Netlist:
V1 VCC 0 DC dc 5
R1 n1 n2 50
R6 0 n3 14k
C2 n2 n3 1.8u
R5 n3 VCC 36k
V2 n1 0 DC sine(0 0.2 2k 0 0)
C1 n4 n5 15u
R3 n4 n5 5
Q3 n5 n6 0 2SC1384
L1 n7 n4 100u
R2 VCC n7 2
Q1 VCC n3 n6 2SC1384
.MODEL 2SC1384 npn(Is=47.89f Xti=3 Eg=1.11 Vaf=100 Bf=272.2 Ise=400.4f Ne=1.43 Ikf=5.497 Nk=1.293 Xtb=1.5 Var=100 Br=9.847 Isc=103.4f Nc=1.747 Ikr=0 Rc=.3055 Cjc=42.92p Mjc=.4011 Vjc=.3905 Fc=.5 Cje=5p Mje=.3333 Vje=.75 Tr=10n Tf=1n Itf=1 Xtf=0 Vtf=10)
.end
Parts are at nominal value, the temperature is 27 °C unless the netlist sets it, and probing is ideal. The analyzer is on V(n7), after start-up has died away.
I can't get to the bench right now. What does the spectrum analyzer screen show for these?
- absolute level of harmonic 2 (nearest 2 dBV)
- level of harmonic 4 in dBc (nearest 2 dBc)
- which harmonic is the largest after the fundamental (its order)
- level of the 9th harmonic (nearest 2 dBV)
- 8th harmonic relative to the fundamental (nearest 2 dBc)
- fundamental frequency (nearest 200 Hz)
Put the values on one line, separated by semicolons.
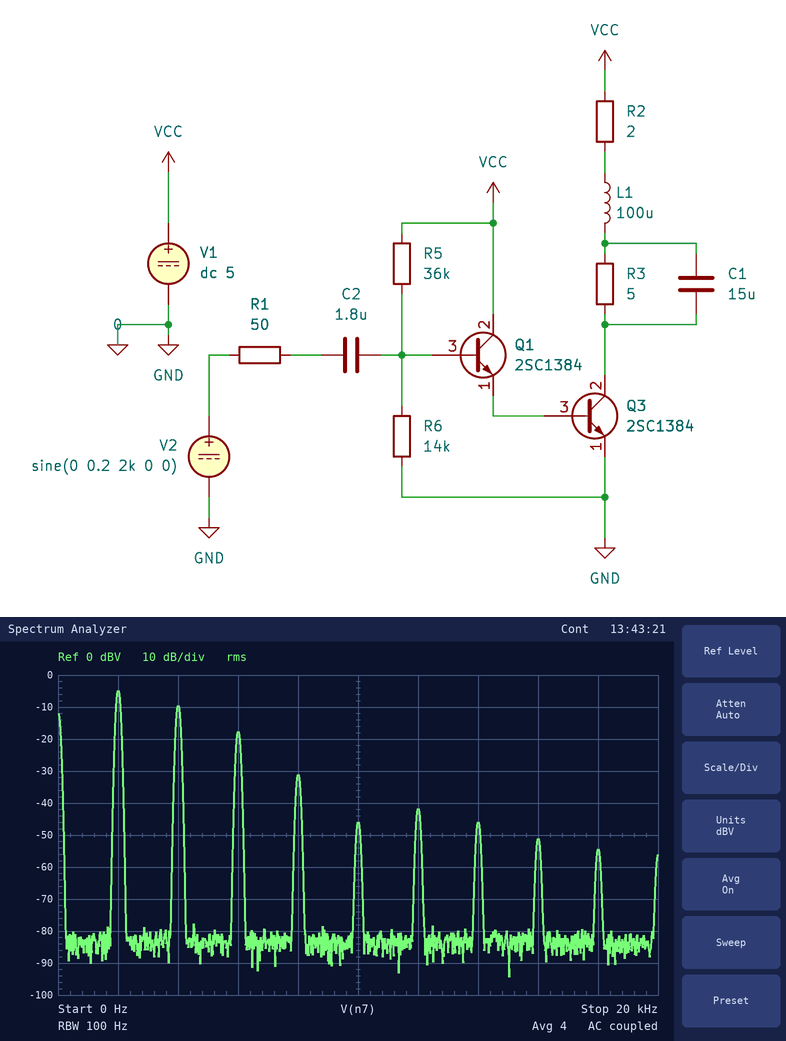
-10 dBV; -26 dBc; 2; -54 dBV; -46 dBc; 2.0 kHz
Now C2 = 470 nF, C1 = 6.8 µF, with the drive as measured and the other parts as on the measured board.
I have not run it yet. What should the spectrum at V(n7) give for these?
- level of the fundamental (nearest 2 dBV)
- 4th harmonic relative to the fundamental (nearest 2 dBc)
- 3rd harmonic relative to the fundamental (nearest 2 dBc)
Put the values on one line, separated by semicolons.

-6 dBV; -30 dBc; -14 dBc
